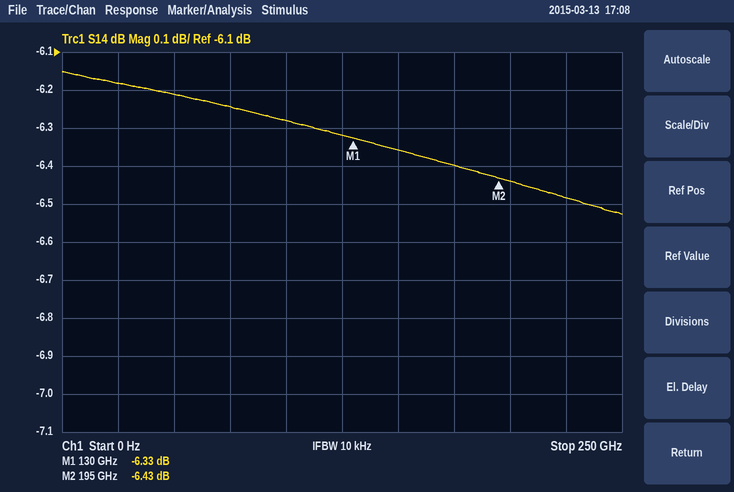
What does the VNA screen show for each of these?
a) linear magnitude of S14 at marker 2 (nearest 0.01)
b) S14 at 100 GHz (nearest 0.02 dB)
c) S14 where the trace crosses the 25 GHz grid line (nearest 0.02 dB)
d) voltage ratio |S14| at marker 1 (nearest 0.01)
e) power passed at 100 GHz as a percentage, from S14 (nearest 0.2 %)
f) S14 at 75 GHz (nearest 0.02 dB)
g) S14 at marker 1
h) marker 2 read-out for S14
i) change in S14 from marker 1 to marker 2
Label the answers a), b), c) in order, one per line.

a) 0.48
b) -6.28 dB
c) -6.18 dB
d) 0.48
e) 23.6 %
f) -6.24 dB
g) -6.33 dB
h) -6.43 dB
i) -0.10 dB
